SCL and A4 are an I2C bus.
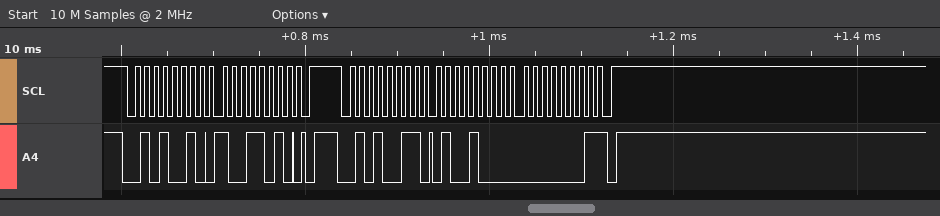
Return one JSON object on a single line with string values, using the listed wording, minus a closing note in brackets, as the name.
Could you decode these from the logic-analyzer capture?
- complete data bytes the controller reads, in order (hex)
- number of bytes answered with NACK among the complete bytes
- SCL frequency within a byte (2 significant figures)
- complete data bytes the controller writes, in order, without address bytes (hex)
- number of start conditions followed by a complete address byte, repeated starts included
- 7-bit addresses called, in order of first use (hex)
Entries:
{"complete data bytes the controller reads, in order": "48 01", "number of bytes answered with NACK among the complete bytes": "1", "SCL frequency within a byte": "100 kHz", "complete data bytes the controller writes, in order, without address bytes": "9A", "number of start conditions followed by a complete address byte, repeated starts included": "2", "7-bit addresses called, in order of first use": "0x29"}
